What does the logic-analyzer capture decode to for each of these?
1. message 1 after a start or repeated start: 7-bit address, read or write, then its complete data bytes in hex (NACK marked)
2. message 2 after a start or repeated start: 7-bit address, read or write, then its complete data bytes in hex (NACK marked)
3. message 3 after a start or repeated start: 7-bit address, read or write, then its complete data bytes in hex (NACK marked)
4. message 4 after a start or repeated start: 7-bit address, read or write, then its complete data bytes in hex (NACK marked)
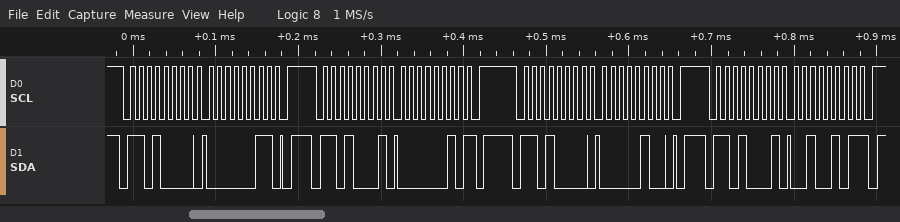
0x68 write: 03
0x68 read: 02 NACK
0x68 write: 04
0x68 read: 25 NACK
